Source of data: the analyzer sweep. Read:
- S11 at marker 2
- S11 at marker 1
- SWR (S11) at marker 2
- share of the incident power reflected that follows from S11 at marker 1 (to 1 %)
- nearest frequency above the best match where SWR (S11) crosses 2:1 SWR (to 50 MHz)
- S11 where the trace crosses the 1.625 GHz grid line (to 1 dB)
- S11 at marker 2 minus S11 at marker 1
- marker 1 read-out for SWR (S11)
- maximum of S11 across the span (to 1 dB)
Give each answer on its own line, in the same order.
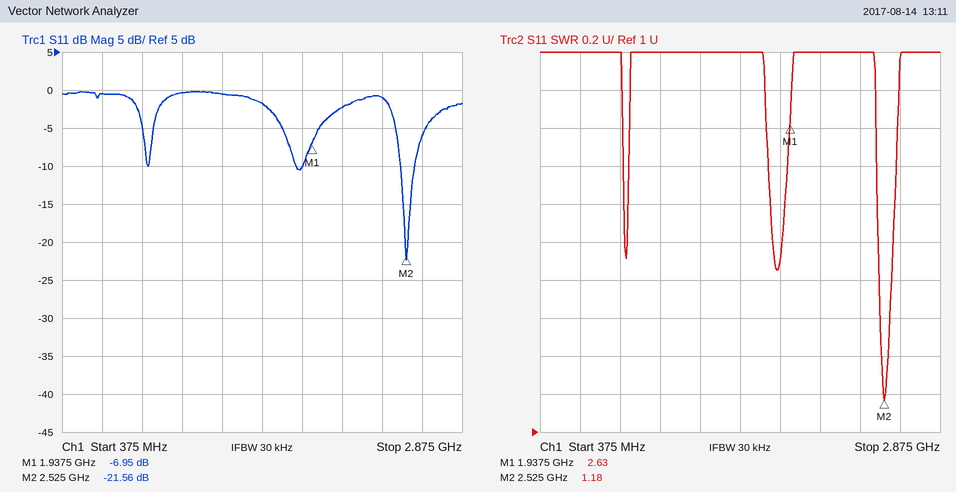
-21.56 dB
-6.95 dB
1.18
20 %
2.60 GHz
-2 dB
-14.61 dB
2.63
0 dB
